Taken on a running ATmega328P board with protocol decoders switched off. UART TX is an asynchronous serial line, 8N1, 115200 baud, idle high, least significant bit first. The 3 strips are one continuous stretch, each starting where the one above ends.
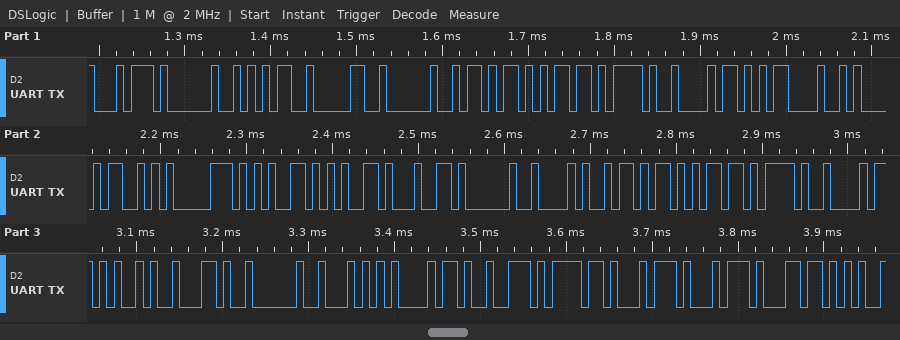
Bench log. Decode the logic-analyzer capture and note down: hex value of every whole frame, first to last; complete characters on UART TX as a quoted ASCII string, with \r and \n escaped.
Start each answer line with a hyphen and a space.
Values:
- 74 20 35 30 20 6B 6D 2F 68 0D 0A 53 70 65 65 64 20 28 6B 6D 2F 68 29 2C 20 54 68 72 6F 74 74 6C
- "t 50 km/h\r\nSpeed (km/h), Throttl"
